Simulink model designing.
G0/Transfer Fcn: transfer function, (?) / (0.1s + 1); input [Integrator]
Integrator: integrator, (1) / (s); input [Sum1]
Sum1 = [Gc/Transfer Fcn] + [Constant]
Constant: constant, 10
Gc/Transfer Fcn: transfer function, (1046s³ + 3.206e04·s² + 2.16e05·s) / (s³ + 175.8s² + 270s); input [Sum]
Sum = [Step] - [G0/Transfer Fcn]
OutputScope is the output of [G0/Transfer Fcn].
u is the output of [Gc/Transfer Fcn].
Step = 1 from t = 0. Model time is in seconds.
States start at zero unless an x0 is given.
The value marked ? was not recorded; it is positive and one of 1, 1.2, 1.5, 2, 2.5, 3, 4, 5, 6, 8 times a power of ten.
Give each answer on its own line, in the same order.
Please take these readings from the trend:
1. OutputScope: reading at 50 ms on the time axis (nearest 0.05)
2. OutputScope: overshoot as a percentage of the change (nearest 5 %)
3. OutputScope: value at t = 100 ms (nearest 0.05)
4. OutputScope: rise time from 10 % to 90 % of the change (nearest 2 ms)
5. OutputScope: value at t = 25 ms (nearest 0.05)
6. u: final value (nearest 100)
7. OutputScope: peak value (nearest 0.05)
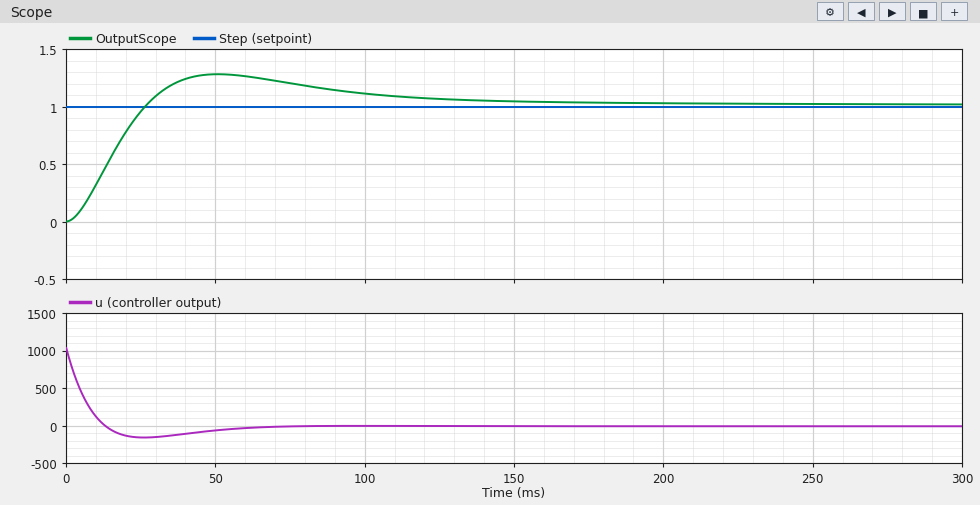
1.30
25 %
1.10
18 ms
0.95
0
1.30
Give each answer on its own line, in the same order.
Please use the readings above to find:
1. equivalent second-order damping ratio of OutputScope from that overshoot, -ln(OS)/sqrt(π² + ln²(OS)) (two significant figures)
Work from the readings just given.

0.40
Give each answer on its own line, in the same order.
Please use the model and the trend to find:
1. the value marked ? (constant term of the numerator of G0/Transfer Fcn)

1
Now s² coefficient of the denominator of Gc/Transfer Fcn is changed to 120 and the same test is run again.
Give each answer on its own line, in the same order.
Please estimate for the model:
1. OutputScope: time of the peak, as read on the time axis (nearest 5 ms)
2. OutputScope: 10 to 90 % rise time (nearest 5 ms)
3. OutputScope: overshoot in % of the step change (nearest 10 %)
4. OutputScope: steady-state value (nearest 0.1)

40 ms
15 ms
30 %
1.0
